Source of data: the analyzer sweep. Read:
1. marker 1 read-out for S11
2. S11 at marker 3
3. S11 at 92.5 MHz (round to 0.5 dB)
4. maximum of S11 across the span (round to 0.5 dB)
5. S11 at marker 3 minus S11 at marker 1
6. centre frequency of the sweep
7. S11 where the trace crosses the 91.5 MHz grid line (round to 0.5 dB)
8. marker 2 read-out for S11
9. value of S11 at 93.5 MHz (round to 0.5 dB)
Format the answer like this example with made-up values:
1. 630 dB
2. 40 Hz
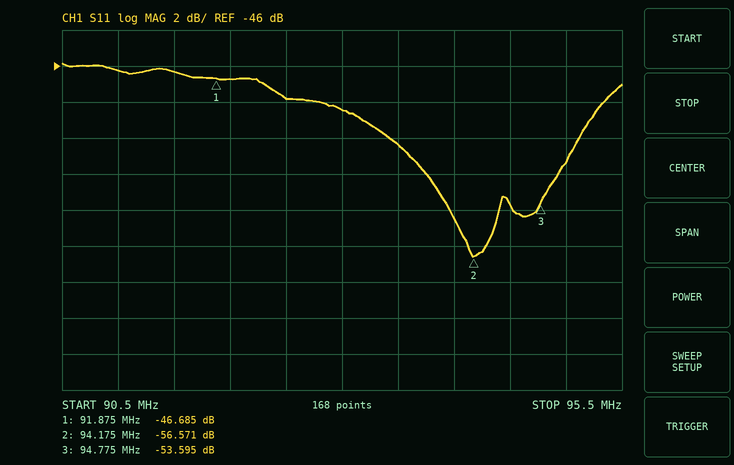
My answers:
1. -46.685 dB
2. -53.595 dB
3. -48.0 dB
4. -46.0 dB
5. -6.910 dB
6. 93 MHz
7. -46.5 dB
8. -56.571 dB
9. -50.5 dB
